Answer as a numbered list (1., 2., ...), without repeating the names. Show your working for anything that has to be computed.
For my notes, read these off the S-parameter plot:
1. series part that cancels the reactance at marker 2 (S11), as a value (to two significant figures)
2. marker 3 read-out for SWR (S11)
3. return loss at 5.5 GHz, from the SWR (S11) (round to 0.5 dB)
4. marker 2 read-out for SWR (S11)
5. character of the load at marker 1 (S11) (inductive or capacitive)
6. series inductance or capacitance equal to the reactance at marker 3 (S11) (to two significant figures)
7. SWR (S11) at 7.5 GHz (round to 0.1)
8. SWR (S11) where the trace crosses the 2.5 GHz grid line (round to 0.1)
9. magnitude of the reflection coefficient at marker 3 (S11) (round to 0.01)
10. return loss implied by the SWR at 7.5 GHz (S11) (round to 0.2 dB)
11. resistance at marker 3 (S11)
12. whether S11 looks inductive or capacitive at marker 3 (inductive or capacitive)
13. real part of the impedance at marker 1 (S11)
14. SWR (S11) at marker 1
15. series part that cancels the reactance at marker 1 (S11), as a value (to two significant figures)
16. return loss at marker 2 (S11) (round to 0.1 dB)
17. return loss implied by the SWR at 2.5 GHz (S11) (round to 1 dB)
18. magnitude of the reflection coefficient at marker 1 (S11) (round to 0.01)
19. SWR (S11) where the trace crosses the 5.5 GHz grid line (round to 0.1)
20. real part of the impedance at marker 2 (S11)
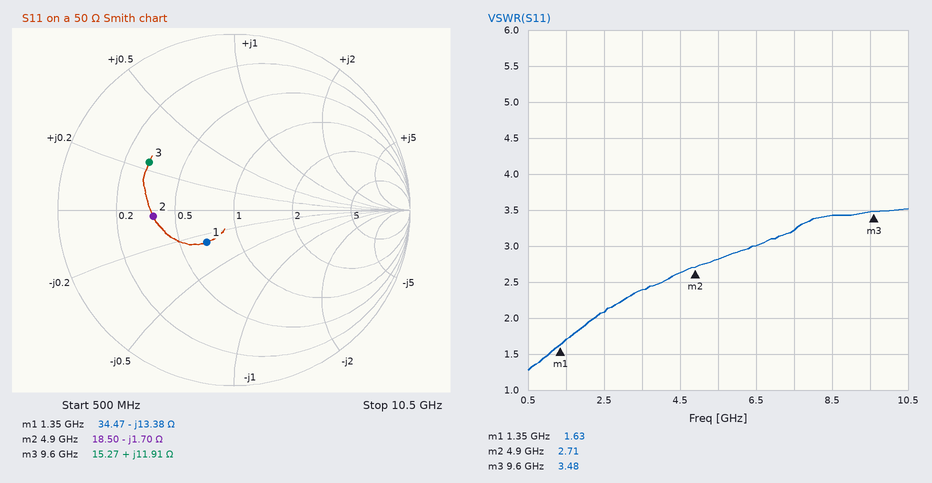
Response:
1. L = 1.7 Ω/(2π × 4.9 GHz) ≈ 55 pH
2. 3.48
3. −20 log10((2.8 − 1)/(2.8 + 1)) ≈ 6.5 dB
4. 2.71
5. capacitive
6. L = 11.91 Ω/(2π × 9.6 GHz) ≈ 197 pH, so 200 pH to two significant figures
7. 3.2
8. 2.1
9. 0.55
10. −20 log10((3.2 − 1)/(3.2 + 1)) ≈ 5.6 dB
11. 15.27 Ω
12. inductive
13. 34.47 Ω
14. 1.63
15. L = 13.38 Ω/(2π × 1.35 GHz) ≈ 1.6 nH
16. 6.7 dB
17. −20 log10((2.1 − 1)/(2.1 + 1)) ≈ 9 dB
18. 0.24
19. 2.8
20. 18.50 Ω
